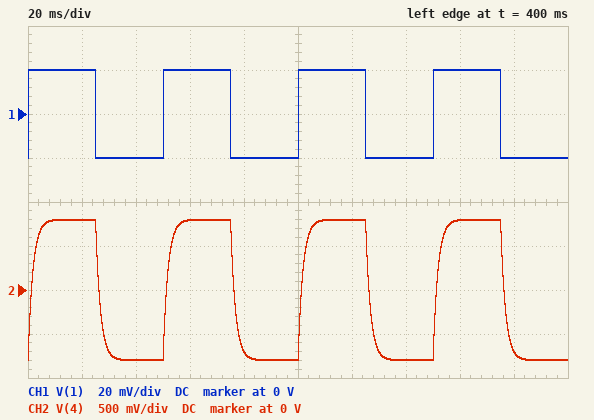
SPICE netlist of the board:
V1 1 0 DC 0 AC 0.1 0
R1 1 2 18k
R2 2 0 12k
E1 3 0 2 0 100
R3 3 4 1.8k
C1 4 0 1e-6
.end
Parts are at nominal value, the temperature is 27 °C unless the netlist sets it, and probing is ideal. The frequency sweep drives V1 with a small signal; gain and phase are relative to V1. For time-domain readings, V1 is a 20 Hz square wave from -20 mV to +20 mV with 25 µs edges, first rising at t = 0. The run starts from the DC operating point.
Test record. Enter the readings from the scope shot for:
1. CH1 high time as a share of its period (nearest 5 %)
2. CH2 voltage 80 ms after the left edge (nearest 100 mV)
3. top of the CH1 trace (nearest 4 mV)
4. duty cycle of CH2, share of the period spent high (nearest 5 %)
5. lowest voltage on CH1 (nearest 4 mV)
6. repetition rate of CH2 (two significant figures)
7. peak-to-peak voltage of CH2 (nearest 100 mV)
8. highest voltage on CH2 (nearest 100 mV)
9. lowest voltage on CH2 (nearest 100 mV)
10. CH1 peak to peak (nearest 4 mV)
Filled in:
50 %
-700 mV
20 mV
50 %
-20 mV
20 Hz
1.6 V
800 mV
-800 mV
40 mV
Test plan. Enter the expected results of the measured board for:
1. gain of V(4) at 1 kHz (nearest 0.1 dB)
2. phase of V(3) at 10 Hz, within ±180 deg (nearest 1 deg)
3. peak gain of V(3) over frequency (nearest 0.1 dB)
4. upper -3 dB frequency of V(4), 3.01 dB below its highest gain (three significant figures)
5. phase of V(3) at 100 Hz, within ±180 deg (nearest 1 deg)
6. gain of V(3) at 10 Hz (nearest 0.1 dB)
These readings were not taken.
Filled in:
10.9 dB
0 deg
32.0 dB
88.4 Hz
0 deg
32.0 dB
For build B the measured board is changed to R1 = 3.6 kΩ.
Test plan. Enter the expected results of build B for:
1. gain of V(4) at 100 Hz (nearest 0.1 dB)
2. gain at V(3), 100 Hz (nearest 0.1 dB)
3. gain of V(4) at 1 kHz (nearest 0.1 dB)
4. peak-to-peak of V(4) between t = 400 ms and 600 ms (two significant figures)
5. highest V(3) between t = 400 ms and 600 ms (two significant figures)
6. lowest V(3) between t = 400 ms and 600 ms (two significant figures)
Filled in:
34.1 dB
37.7 dB
16.6 dB
3.1 V
1.5 V
-1.5 V
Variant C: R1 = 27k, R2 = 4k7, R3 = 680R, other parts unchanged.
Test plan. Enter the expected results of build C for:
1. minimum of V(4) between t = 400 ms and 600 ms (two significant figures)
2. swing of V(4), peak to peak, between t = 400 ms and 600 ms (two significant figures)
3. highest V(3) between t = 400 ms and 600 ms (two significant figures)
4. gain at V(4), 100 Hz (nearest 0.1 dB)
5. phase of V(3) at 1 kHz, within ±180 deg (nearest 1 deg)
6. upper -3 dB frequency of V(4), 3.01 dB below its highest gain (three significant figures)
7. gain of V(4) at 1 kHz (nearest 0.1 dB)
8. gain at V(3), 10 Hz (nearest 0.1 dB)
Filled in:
-300 mV
590 mV
300 mV
22.7 dB
0 deg
234 Hz
10.6 dB
23.4 dB
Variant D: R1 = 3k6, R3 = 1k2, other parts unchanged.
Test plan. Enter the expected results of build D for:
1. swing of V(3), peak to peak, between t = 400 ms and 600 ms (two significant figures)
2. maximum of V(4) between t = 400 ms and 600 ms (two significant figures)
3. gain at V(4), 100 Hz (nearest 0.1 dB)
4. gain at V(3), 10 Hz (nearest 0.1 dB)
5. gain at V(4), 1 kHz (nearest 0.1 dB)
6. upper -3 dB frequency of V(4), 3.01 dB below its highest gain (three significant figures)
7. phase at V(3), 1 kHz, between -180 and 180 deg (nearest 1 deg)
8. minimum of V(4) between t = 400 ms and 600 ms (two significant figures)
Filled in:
3.1 V
1.5 V
35.8 dB
37.7 dB
20.1 dB
133 Hz
0 deg
-1.5 V
